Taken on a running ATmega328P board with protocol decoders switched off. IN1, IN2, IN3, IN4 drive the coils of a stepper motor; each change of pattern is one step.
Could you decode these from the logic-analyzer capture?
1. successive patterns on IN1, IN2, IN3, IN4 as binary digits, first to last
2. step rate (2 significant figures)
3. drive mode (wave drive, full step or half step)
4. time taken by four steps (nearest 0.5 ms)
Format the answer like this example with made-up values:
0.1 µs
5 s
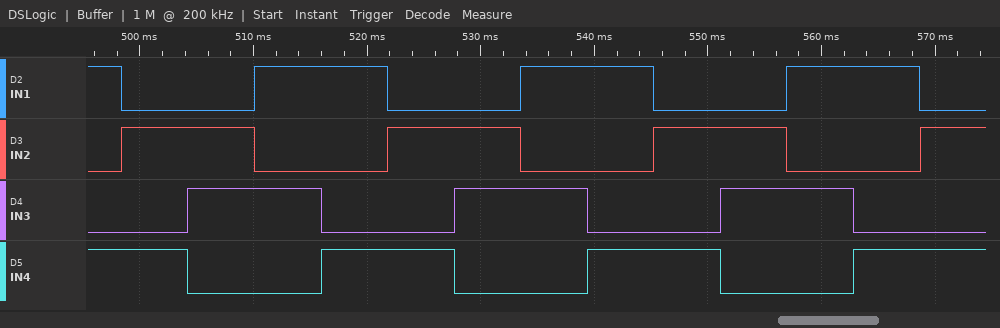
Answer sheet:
1001 0101 0110 1010 1001 0101 0110 1010 1001 0101 0110 1010 1001 0101
170 steps/s
full step
23.5 ms
